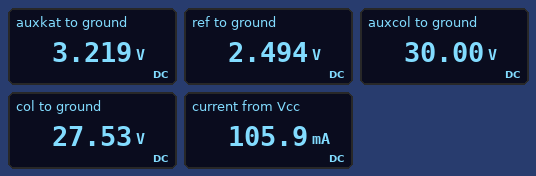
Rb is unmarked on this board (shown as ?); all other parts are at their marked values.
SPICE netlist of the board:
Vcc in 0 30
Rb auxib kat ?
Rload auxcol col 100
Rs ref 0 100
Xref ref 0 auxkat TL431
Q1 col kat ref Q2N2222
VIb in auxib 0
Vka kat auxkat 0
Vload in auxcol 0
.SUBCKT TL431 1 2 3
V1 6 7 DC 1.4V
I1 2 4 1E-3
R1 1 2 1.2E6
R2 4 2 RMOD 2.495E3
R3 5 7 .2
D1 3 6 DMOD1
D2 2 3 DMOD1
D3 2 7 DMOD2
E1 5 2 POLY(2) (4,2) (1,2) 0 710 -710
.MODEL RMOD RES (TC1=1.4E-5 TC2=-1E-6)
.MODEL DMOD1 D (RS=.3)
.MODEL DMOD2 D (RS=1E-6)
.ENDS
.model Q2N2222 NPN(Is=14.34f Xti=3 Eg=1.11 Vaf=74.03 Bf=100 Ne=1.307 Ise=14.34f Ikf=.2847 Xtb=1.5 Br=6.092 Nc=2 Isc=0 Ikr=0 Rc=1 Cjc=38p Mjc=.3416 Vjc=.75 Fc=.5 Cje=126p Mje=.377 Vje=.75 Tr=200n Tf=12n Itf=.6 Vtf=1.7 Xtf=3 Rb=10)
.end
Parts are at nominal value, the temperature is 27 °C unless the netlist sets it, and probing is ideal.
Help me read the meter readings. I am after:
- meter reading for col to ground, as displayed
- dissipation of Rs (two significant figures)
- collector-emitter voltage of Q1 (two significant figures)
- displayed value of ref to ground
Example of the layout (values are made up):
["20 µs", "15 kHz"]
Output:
["27.53 V", "62 mW", "25 V", "2.494 V"]
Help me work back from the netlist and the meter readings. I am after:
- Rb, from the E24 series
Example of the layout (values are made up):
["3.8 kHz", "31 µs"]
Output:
["330 Ω"]
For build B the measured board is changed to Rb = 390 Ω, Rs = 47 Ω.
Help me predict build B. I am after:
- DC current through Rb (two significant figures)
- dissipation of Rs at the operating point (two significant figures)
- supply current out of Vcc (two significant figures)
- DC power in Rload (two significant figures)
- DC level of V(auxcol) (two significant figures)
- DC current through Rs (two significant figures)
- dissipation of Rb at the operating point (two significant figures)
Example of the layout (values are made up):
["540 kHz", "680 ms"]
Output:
["69 mA", "130 mW", "120 mA", "280 mW", "30 V", "53 mA", "1.8 W"]
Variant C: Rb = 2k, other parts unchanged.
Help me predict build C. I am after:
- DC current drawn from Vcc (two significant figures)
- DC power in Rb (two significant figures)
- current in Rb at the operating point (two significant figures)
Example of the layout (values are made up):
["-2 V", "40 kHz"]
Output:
["38 mA", "360 mW", "13 mA"]
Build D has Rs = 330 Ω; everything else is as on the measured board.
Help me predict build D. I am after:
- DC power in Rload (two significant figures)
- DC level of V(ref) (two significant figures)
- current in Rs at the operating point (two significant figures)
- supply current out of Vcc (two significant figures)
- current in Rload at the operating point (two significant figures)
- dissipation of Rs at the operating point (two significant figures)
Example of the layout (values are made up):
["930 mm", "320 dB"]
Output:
["5.6 mW", "2.5 V", "7.6 mA", "89 mA", "7.5 mA", "19 mW"]
